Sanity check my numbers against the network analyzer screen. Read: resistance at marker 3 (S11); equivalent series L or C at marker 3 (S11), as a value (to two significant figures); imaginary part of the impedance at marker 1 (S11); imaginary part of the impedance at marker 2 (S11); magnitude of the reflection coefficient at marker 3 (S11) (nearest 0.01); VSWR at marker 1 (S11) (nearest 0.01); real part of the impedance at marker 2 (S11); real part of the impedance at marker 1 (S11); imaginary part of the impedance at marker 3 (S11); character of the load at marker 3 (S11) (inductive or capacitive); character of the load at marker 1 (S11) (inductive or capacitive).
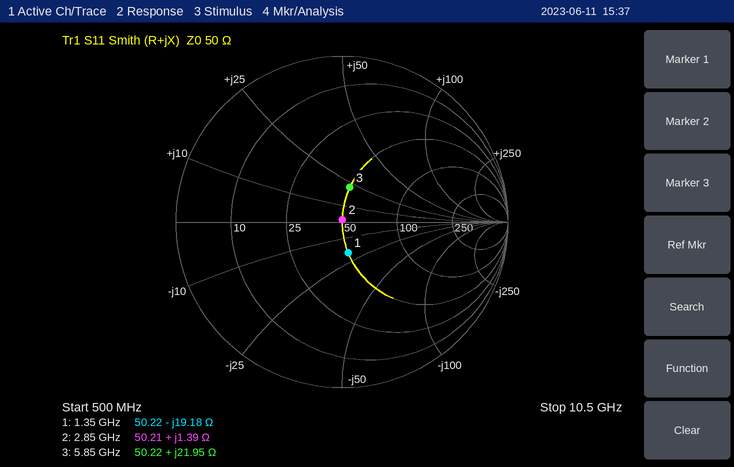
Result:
50.22 Ω
600 pH
-19.18 Ω
+1.39 Ω
0.21
1.46
50.21 Ω
50.22 Ω
+21.95 Ω
inductive
capacitive
